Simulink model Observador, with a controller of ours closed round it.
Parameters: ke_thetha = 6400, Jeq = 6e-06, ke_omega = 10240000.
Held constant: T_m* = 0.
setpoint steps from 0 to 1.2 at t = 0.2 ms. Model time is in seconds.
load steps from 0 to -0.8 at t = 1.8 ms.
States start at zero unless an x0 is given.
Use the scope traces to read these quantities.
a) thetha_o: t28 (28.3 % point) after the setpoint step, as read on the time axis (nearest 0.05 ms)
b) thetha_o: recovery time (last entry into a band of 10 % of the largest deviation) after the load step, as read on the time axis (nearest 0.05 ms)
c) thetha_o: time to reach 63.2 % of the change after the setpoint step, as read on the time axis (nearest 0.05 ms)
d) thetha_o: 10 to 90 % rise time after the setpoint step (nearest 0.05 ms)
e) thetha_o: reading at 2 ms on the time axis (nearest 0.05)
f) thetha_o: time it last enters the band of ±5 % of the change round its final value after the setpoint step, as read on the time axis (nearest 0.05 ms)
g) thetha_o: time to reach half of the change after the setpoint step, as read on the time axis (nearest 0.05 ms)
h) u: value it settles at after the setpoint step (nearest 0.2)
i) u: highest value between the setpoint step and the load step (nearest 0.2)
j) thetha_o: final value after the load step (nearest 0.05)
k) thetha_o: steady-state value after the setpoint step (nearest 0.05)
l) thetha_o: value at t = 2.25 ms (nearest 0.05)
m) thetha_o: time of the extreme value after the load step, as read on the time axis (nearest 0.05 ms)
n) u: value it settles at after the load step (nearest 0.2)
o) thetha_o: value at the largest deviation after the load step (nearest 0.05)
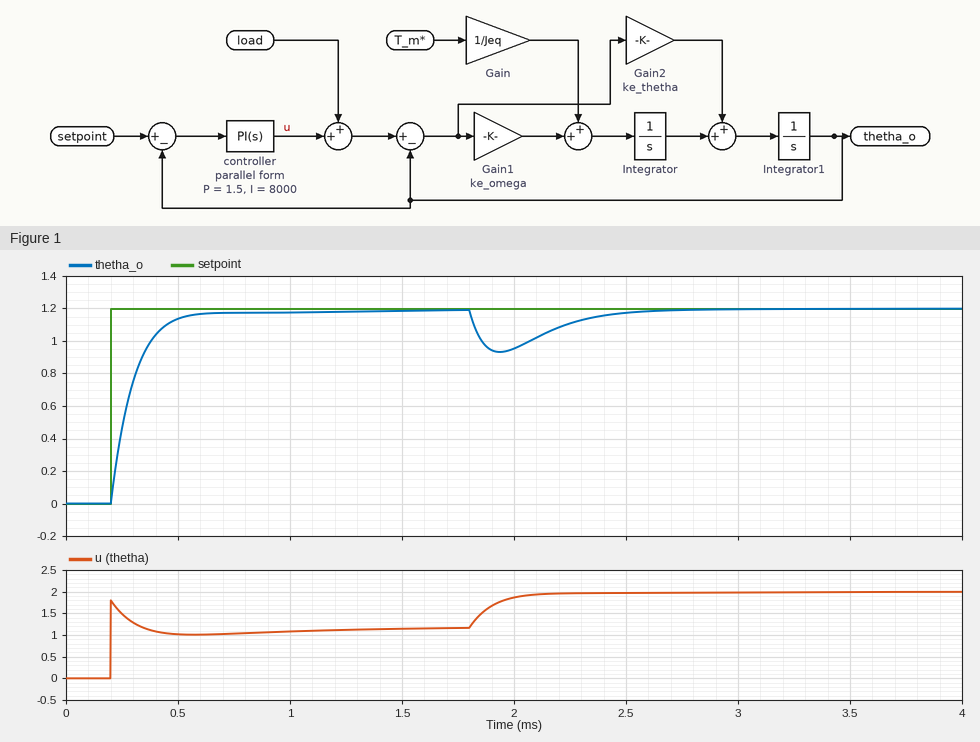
0.25 ms
2.50 ms
0.30 ms
0.20 ms
0.95
0.50 ms
0.25 ms
1.2
1.8
1.20
1.20
1.10
1.95 ms
2.0
0.95
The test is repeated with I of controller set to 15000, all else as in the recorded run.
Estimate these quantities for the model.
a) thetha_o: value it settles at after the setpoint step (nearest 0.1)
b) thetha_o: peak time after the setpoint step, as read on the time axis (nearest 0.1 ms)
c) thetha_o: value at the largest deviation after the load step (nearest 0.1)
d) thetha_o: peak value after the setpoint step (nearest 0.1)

1.2
0.5 ms
1.0
1.3
